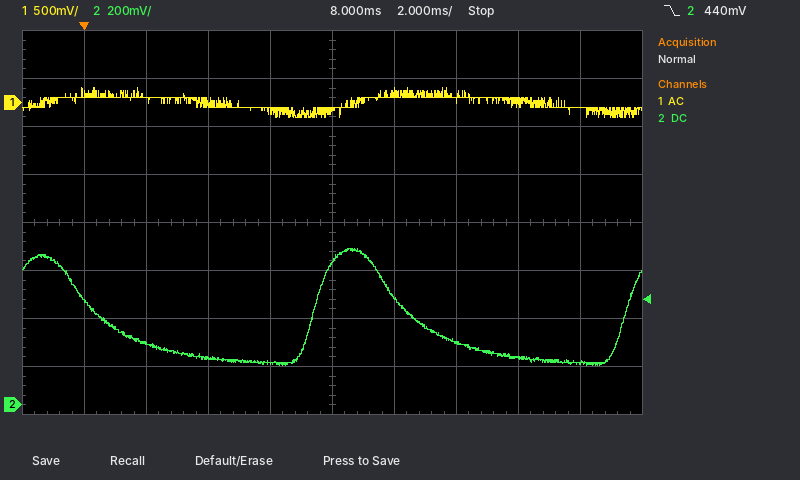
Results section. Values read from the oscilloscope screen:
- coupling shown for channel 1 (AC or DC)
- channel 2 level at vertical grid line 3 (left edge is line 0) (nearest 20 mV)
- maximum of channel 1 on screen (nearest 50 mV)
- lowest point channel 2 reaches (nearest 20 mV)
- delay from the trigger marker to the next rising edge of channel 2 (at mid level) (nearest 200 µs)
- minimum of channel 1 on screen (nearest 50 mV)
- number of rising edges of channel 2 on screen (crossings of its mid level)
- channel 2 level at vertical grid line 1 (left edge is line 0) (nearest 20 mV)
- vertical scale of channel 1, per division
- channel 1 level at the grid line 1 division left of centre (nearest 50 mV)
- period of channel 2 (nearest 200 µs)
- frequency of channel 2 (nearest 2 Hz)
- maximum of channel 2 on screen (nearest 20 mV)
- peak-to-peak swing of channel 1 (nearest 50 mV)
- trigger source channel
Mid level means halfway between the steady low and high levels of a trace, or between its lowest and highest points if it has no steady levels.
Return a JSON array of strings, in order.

["AC", "200 mV", "150 mV", "160 mV", "7.4 ms", "-150 mV", "2", "440 mV", "500 mV", "-100 mV", "10.0 ms", "100 Hz", "660 mV", "300 mV", "channel 2"]
